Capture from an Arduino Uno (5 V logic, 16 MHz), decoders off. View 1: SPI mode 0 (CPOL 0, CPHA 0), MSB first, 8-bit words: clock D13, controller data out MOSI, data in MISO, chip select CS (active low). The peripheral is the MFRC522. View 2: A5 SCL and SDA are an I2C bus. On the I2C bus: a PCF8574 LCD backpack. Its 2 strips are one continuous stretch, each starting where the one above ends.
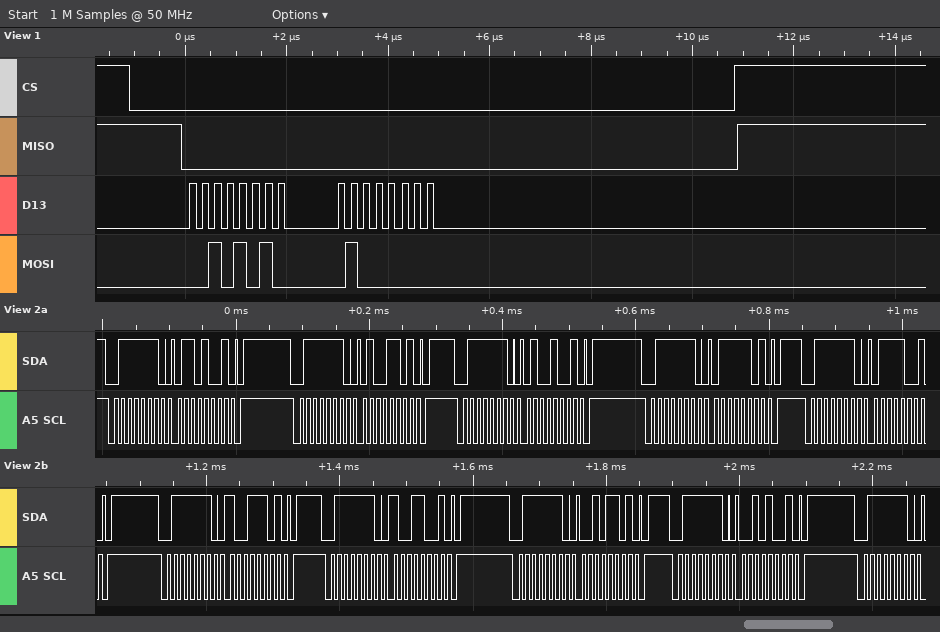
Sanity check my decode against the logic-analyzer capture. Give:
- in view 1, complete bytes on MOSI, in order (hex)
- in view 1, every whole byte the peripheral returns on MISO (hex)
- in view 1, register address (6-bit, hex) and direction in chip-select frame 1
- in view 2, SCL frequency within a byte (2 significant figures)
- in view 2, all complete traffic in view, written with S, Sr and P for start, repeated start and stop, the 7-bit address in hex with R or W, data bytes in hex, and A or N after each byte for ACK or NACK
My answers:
2A 40
00 00
0x15 write
100 kHz
S 3FW A 69 A P S 3FW A 4D A P S 3FW A 49 A P S 3FW A 7D A P S 3FW A 79 A P S 3FW A 9D A P S 3FW A 99 A P S 3FW A 2D A P S 3FW A 29 A P S 3FW A
